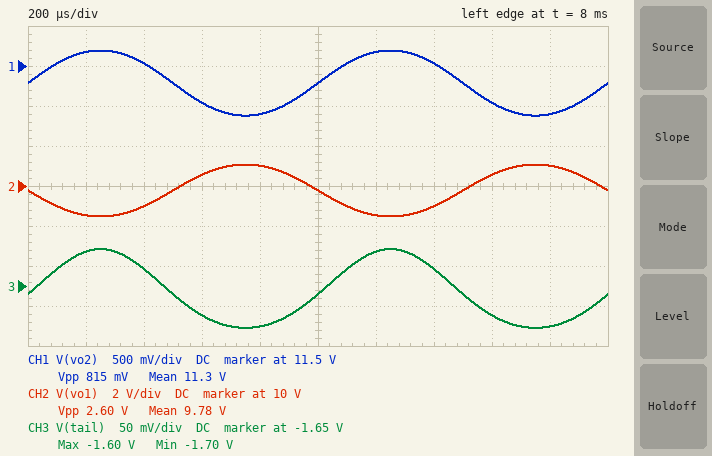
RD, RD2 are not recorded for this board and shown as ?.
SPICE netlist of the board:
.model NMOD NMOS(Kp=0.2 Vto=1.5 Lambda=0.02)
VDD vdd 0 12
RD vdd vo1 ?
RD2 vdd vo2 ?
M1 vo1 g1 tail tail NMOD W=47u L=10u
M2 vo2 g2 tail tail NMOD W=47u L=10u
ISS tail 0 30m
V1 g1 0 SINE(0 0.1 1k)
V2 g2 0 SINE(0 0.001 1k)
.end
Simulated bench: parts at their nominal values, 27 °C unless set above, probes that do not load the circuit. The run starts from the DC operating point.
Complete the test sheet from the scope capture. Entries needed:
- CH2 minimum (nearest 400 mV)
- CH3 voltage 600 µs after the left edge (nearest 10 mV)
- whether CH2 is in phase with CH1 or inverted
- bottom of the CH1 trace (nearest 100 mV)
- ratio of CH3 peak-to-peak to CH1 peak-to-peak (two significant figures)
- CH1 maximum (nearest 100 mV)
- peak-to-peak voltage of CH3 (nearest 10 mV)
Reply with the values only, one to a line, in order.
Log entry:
8.4 V
-1.69 V
inverted
10.9 V
0.12
11.7 V
100 mV
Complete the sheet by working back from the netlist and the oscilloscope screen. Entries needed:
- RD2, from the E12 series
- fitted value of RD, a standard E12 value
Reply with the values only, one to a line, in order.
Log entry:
47 Ω
150 Ω
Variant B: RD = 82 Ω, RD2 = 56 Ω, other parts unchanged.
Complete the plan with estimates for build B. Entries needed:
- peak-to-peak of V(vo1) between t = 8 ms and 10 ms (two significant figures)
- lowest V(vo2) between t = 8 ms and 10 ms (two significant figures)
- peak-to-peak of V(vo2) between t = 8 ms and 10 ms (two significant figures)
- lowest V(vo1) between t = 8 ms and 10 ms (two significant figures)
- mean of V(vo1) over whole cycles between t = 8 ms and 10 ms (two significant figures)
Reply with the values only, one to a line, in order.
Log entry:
1.4 V
11 V
980 mV
10 V
11 V
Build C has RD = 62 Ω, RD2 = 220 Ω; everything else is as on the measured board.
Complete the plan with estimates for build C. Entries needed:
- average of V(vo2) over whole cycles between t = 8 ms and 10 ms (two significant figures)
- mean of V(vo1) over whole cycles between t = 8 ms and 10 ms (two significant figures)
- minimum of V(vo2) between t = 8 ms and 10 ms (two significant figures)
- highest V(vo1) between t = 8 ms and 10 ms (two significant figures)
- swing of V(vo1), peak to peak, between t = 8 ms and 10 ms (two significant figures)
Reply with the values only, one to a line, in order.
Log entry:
8.8 V
11 V
6.9 V
12 V
1.1 V
